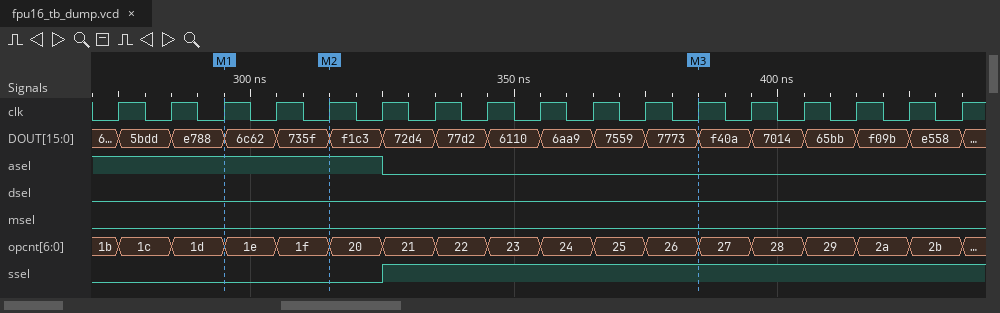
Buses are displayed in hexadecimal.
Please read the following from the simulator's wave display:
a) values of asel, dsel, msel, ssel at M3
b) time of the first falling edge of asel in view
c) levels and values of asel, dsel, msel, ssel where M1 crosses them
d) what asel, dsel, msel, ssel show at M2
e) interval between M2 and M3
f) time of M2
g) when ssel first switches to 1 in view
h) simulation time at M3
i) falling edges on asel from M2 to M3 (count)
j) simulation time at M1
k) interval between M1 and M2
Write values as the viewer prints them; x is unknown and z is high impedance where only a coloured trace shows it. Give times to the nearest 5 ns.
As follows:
asel=0, dsel=0, msel=0, ssel=1
325 ns
asel=1, dsel=0, msel=0, ssel=0
asel=1, dsel=0, msel=0, ssel=0
70 ns
315 ns
325 ns
385 ns
1
295 ns
20 ns
